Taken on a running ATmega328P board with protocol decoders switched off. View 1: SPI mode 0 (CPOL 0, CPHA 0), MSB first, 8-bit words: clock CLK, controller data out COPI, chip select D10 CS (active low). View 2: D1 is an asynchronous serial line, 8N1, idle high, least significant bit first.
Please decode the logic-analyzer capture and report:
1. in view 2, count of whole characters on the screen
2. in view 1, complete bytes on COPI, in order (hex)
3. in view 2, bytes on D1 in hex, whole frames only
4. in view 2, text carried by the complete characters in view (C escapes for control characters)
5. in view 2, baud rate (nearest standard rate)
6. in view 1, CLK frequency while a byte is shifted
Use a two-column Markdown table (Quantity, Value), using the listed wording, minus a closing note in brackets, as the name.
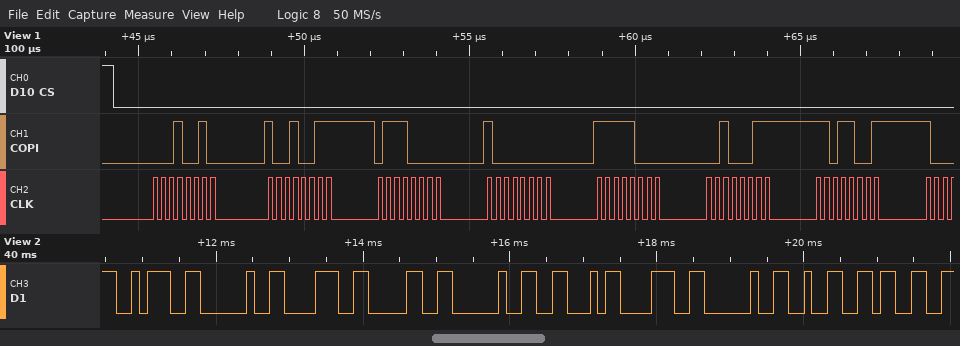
| Quantity | Value |
|---|---|
| in view 2, count of whole characters on the screen | 10 |
| in view 1, complete bytes on COPI, in order | 12 93 70 80 F8 23 D9 |
| in view 2, bytes on D1 in hex, whole frames only | 3A 20 38 30 20 46 38 20 32 33 |
| in view 2, text carried by the complete characters in view | ": 80 F8 23" |
| in view 2, baud rate | 9600 baud |
| in view 1, CLK frequency while a byte is shifted | 4 MHz |
